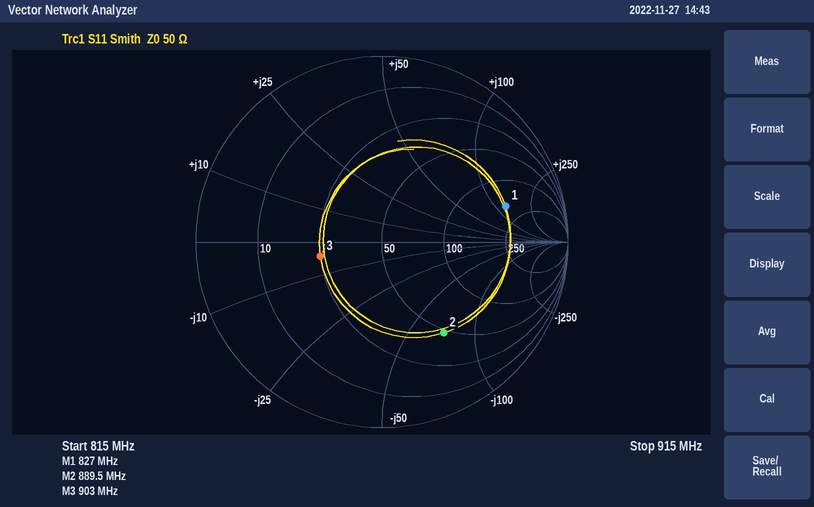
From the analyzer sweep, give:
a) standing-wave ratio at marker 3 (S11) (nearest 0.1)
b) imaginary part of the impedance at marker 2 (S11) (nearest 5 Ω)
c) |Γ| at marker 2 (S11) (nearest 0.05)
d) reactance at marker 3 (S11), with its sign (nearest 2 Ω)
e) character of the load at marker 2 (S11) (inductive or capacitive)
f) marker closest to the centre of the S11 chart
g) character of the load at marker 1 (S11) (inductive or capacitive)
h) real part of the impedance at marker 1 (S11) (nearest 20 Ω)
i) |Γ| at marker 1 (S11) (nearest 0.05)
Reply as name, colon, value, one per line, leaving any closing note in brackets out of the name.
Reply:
standing-wave ratio at marker 3 (S11): 2.0
imaginary part of the impedance at marker 2 (S11): -70 Ω
|Γ| at marker 2 (S11): 0.60
reactance at marker 3 (S11), with its sign: -4 Ω
character of the load at marker 2 (S11): capacitive
marker closest to the centre of the S11 chart: marker 3
character of the load at marker 1 (S11): inductive
real part of the impedance at marker 1 (S11): 180 Ω
|Γ| at marker 1 (S11): 0.70
